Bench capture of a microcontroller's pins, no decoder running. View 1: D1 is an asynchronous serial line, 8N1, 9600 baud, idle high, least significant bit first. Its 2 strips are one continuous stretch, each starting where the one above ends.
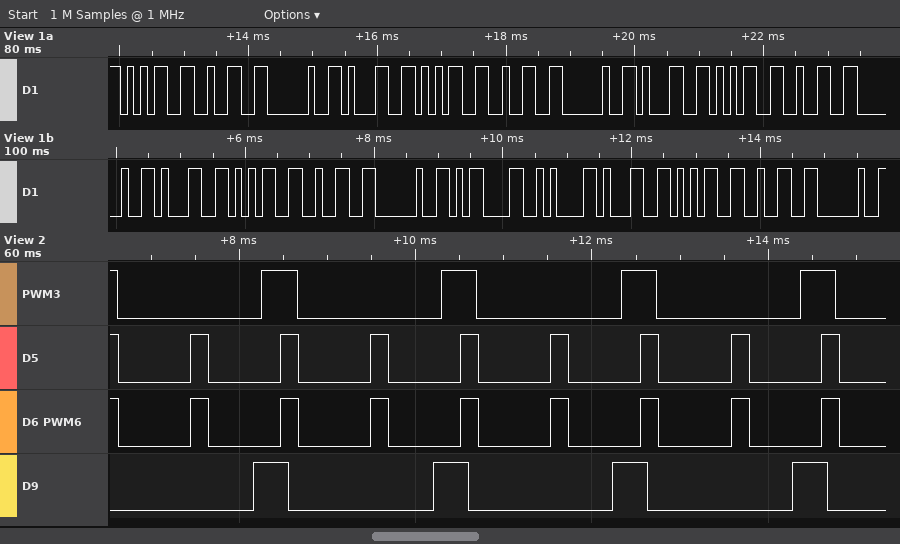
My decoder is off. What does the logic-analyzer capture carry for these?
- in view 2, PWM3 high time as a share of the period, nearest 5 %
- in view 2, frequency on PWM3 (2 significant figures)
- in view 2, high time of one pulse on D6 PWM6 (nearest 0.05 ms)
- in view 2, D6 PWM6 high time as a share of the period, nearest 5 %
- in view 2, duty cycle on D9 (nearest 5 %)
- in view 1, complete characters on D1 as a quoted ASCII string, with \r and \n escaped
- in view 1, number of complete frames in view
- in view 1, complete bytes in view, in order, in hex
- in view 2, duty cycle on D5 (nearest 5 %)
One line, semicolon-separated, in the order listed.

20 %; 490 Hz; 0.20 ms; 20 %; 20 %; "52 152 152 152 \r\n152 "; 21; 35 32 20 31 35 32 20 31 35 32 20 31 35 32 20 0D 0A 31 35 32 20; 20 %
